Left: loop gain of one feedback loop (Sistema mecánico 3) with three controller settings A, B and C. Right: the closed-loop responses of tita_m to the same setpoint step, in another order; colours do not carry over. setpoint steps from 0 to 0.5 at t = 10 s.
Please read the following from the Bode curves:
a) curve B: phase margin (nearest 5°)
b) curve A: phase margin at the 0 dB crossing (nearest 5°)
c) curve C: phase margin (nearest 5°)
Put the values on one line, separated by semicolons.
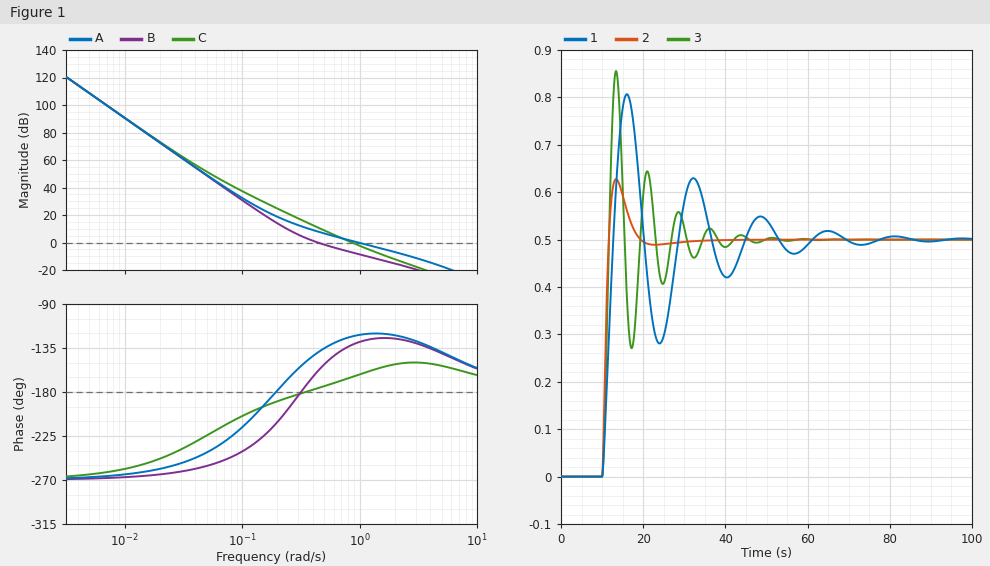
20°; 60°; 15°
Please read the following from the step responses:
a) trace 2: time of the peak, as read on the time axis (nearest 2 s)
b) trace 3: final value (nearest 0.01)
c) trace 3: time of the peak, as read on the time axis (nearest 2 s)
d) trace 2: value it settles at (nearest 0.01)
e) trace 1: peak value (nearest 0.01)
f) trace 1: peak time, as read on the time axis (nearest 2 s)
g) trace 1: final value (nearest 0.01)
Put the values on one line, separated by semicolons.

14 s; 0.50; 14 s; 0.50; 0.81; 16 s; 0.50
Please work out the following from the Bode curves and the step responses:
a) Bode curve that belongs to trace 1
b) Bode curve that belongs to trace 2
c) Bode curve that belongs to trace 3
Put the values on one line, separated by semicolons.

B; A; C
